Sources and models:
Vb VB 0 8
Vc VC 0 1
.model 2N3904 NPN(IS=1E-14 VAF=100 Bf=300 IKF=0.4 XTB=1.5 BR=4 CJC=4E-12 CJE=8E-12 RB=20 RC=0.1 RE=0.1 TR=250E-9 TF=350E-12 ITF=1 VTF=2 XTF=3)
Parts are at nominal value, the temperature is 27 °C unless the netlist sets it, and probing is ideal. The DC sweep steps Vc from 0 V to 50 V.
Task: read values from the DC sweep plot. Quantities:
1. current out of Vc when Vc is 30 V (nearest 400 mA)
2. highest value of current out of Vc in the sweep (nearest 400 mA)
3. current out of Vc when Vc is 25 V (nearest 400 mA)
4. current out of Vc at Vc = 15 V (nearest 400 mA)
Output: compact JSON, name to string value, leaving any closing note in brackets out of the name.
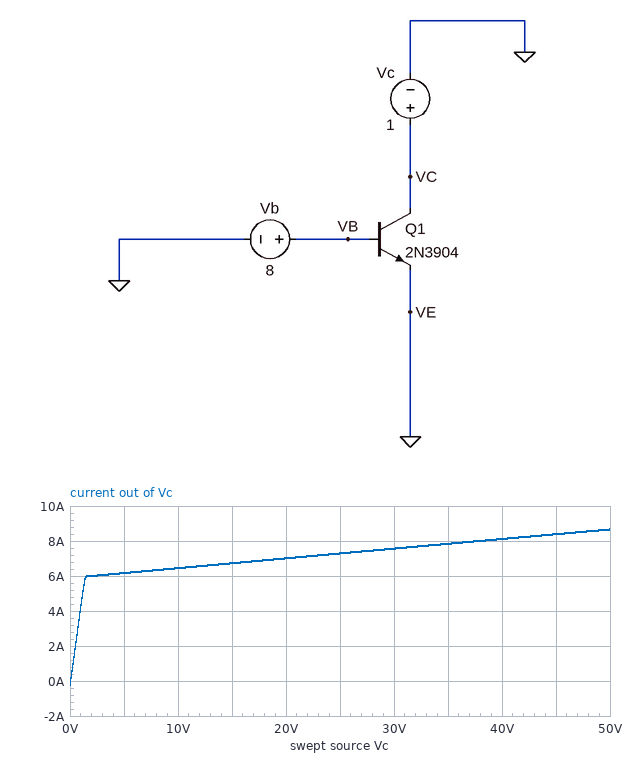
{"current out of Vc when Vc is 30 V": "7.6 A", "highest value of current out of Vc in the sweep": "8.8 A", "current out of Vc when Vc is 25 V": "7.2 A", "current out of Vc at Vc = 15 V": "6.8 A"}
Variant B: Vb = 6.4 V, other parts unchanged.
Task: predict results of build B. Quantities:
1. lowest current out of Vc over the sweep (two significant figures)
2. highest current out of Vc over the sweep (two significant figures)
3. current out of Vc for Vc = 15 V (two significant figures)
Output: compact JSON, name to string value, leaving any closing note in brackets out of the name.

{"lowest current out of Vc over the sweep": "-170 mA", "highest current out of Vc over the sweep": "7.5 A", "current out of Vc for Vc = 15 V": "5.9 A"}
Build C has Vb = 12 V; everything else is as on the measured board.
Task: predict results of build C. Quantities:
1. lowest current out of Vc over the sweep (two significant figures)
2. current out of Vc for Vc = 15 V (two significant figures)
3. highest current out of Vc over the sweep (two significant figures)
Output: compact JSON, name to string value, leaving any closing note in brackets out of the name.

{"lowest current out of Vc over the sweep": "-320 mA", "current out of Vc for Vc = 15 V": "8.5 A", "highest current out of Vc over the sweep": "11 A"}
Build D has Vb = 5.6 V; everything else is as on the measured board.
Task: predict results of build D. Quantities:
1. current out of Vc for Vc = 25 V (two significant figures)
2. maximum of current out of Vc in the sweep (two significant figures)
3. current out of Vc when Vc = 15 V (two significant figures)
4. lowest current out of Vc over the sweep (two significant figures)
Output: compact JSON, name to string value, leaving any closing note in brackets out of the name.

{"current out of Vc for Vc = 25 V": "5.8 A", "maximum of current out of Vc in the sweep": "6.9 A", "current out of Vc when Vc = 15 V": "5.4 A", "lowest current out of Vc over the sweep": "-140 mA"}
